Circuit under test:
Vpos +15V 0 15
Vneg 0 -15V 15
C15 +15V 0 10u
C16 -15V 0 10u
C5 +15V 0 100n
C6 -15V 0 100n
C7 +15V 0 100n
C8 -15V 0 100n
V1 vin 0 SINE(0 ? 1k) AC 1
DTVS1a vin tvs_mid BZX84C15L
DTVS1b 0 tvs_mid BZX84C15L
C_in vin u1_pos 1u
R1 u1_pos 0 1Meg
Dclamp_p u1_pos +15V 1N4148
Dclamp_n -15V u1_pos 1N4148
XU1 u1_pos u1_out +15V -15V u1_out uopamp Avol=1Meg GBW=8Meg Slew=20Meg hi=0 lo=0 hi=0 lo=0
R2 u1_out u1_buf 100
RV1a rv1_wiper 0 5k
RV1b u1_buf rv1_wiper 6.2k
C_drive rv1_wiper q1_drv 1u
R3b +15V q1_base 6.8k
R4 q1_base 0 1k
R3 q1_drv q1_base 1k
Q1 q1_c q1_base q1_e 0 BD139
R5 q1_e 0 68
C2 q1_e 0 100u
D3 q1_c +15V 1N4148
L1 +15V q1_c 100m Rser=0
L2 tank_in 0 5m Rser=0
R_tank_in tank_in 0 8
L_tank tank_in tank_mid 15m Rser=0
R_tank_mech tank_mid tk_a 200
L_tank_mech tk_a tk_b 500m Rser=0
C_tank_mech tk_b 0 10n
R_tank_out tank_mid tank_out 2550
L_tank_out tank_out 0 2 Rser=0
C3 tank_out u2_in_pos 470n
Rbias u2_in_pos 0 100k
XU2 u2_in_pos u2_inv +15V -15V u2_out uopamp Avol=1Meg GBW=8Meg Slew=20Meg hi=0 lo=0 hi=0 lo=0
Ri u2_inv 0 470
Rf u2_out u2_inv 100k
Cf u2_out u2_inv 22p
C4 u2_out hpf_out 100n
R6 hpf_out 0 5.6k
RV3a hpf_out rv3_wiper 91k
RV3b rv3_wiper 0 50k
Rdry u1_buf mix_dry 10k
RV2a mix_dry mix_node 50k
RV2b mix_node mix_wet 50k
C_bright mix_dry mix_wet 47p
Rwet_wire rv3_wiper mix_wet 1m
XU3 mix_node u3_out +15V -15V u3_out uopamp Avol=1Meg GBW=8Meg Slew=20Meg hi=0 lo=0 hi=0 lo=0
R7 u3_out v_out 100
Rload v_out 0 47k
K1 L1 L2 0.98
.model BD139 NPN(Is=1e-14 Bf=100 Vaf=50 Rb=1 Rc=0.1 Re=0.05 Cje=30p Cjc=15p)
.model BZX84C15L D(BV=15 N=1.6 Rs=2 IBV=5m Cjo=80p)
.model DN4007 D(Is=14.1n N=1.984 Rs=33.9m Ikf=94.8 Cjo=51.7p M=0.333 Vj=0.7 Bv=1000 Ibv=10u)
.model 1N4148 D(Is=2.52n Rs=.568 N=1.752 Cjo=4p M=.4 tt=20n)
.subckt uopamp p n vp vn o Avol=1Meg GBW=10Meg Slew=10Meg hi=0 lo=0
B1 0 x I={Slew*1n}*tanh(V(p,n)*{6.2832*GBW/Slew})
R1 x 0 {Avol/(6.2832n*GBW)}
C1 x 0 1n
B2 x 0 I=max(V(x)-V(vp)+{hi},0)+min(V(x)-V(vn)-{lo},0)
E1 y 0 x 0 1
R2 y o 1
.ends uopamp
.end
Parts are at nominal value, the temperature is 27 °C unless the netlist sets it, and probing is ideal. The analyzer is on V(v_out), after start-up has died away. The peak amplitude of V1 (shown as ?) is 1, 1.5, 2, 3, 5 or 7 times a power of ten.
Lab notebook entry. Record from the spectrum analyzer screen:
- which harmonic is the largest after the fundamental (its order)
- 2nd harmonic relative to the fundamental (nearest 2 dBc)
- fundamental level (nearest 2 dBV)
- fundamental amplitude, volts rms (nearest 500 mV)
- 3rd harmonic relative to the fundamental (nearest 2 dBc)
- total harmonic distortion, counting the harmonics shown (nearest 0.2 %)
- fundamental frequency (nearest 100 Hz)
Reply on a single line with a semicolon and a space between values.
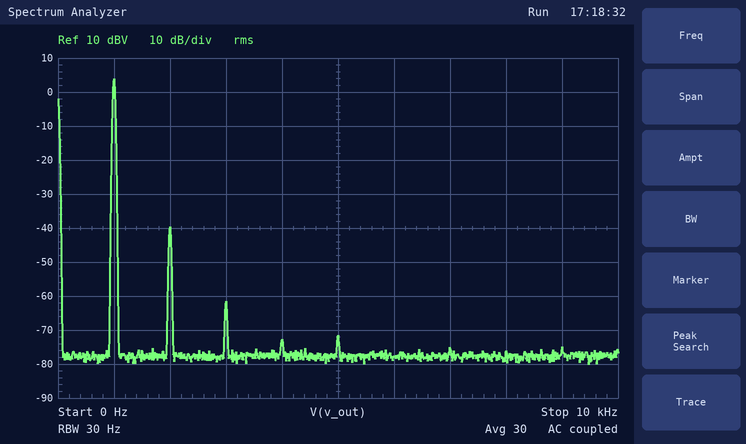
2; -44 dBc; 4 dBV; 1.5 V; -66 dBc; 0.6 %; 1.0 kHz
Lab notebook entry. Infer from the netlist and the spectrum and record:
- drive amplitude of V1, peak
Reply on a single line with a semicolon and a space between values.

200 mV
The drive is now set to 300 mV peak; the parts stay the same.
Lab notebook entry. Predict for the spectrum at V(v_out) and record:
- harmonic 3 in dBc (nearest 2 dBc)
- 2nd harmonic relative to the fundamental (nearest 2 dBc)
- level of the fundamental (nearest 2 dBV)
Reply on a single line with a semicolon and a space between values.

-16 dBc; -40 dBc; 6 dBV
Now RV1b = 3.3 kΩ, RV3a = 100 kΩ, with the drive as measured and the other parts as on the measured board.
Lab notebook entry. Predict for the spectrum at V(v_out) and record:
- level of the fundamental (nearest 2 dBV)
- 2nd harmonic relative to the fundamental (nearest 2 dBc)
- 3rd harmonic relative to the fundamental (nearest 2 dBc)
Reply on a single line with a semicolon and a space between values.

4 dBV; -36 dBc; -14 dBc
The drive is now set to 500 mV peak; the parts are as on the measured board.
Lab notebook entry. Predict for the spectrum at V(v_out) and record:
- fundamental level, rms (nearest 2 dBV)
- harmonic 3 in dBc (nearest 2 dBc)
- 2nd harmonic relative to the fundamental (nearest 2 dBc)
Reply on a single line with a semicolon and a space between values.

6 dBV; -12 dBc; -22 dBc
